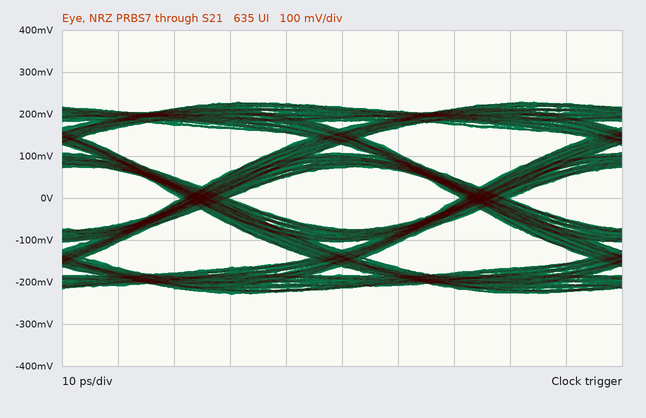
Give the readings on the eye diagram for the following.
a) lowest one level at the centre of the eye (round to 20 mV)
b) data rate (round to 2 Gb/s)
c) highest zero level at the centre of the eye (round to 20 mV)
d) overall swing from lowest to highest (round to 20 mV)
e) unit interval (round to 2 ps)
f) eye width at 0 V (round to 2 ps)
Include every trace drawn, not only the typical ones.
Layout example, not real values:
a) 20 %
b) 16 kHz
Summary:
a) 80 mV
b) 20 Gb/s
c) -80 mV
d) 460 mV
e) 50 ps
f) 42 ps
